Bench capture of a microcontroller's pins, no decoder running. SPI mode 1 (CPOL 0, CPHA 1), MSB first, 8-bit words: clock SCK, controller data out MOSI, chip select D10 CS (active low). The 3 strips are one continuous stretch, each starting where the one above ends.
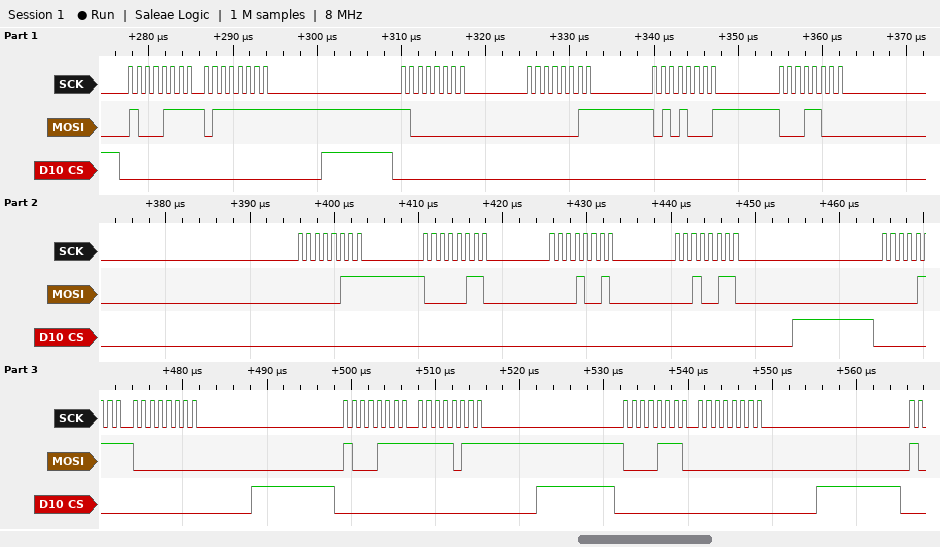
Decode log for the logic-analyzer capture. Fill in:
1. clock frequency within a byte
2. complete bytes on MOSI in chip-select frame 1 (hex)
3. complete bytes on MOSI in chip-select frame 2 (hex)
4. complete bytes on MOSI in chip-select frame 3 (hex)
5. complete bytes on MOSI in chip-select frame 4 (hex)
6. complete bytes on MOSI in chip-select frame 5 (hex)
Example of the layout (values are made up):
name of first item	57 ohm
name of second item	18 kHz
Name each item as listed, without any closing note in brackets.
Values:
clock frequency within a byte	1 MHz
complete bytes on MOSI in chip-select frame 1	8F 7F
complete bytes on MOSI in chip-select frame 2	80 03 51 18 07 06 12 26
complete bytes on MOSI in chip-select frame 3	0F 00
complete bytes on MOSI in chip-select frame 4	8F F7
complete bytes on MOSI in chip-select frame 5	0E 00
